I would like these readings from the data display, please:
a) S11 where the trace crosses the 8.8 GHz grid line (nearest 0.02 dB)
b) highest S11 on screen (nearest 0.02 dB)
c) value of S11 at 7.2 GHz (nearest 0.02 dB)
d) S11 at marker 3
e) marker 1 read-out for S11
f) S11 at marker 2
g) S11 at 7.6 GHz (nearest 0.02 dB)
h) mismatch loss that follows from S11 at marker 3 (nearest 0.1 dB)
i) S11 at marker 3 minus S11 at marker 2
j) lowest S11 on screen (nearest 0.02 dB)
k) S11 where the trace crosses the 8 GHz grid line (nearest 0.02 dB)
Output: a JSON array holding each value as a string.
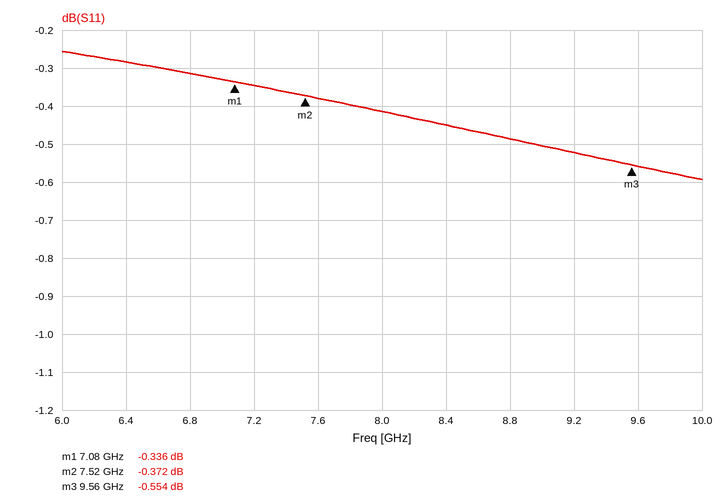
["-0.48 dB", "-0.26 dB", "-0.34 dB", "-0.554 dB", "-0.336 dB", "-0.372 dB", "-0.38 dB", "9.2 dB", "-0.182 dB", "-0.60 dB", "-0.42 dB"]
